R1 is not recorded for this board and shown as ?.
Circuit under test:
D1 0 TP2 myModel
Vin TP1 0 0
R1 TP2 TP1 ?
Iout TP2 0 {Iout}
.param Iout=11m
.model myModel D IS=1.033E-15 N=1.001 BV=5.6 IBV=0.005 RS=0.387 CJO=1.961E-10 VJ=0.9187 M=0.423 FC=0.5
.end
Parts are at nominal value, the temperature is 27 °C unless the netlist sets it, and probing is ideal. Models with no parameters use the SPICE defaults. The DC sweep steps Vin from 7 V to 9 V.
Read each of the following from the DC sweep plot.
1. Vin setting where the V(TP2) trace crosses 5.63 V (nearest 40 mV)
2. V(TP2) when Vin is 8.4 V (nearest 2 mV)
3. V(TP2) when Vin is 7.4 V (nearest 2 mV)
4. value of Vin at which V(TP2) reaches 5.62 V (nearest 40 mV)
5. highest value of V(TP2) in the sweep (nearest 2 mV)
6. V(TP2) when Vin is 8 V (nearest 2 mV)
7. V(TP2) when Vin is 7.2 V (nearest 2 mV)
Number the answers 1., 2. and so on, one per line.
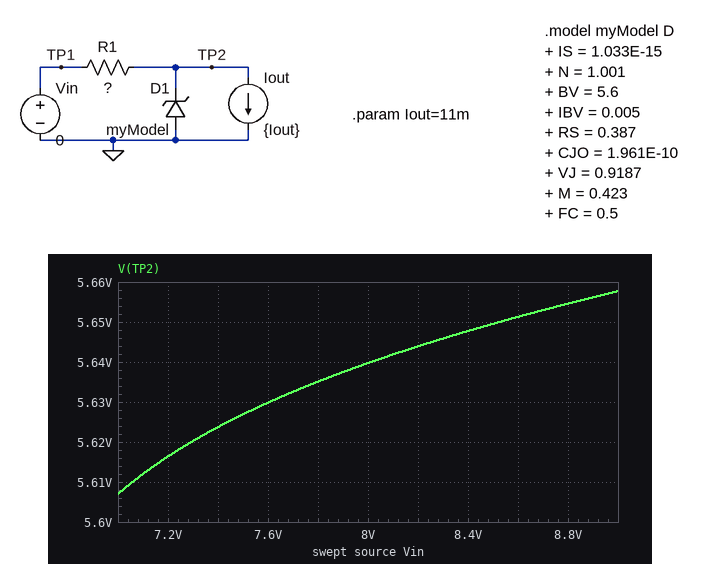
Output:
1. 7.60 V
2. 5.648 V
3. 5.624 V
4. 7.28 V
5. 5.658 V
6. 5.640 V
7. 5.616 V
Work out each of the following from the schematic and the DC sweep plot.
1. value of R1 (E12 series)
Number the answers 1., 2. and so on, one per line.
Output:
1. 82 Ω
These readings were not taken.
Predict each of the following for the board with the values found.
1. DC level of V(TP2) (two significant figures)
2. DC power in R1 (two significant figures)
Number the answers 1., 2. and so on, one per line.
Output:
1. -730 mV
2. 6.6 mW
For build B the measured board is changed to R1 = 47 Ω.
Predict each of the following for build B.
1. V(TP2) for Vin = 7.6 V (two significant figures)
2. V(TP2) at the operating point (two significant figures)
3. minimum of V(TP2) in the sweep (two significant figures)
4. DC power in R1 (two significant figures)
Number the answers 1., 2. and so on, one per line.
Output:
1. 5.7 V
2. -520 mV
3. 5.6 V
4. 5.7 mW
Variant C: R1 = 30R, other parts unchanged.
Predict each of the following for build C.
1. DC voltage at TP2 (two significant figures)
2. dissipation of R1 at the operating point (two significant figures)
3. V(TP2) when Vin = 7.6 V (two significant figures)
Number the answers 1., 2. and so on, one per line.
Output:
1. -330 mV
2. 3.6 mW
3. 5.7 V
